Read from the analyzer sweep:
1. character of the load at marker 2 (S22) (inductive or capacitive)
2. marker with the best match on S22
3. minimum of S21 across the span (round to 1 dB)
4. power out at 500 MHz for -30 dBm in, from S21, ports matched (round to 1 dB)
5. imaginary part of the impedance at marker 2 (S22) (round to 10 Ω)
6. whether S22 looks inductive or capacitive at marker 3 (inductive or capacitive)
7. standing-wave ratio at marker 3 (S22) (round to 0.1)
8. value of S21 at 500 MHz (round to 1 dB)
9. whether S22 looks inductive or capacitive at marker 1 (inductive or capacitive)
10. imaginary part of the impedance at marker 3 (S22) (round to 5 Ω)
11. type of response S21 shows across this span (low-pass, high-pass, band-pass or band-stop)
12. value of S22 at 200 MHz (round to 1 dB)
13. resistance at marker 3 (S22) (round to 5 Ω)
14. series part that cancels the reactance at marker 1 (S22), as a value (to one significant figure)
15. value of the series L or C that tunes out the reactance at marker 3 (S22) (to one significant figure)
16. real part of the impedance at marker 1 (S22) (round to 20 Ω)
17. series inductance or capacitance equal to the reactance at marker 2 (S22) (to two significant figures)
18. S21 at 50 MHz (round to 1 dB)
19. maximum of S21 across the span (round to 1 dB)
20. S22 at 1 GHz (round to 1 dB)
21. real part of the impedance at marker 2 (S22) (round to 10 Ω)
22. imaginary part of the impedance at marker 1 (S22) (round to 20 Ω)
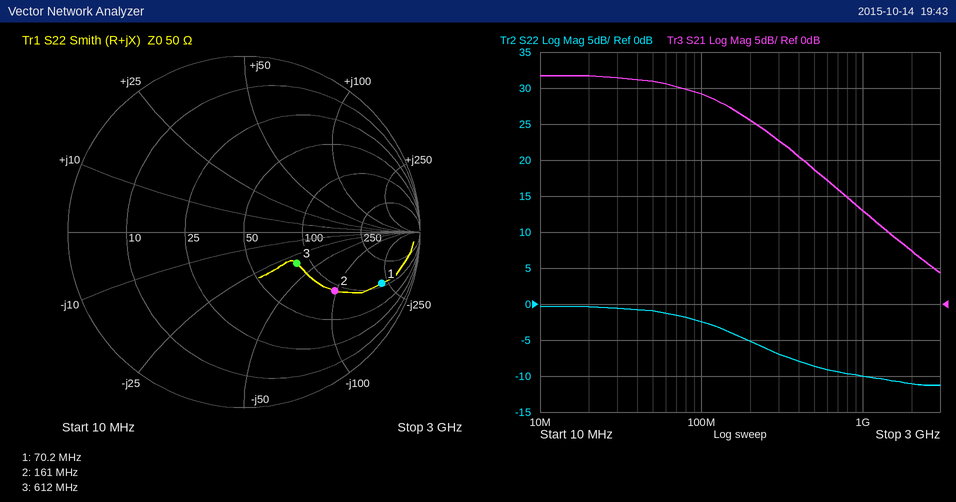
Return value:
capacitive
marker 3
4 dB
-11 dBm
-100 Ω
capacitive
2.1
19 dB
capacitive
-35 Ω
low-pass
-5 dB
85 Ω
500 nH
9 nH
120 Ω
10 pF
31 dB
32 dB
-10 dB
90 Ω
-220 Ω
